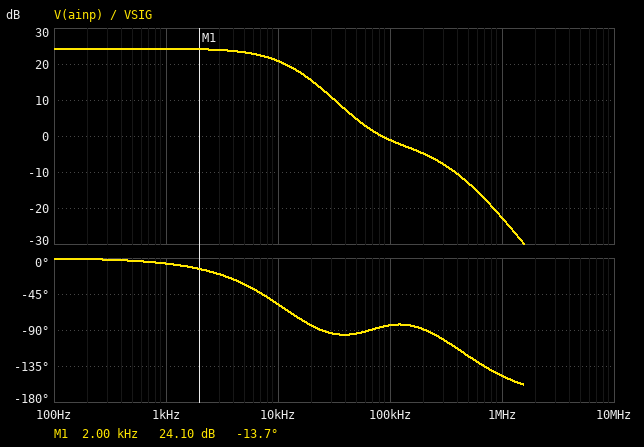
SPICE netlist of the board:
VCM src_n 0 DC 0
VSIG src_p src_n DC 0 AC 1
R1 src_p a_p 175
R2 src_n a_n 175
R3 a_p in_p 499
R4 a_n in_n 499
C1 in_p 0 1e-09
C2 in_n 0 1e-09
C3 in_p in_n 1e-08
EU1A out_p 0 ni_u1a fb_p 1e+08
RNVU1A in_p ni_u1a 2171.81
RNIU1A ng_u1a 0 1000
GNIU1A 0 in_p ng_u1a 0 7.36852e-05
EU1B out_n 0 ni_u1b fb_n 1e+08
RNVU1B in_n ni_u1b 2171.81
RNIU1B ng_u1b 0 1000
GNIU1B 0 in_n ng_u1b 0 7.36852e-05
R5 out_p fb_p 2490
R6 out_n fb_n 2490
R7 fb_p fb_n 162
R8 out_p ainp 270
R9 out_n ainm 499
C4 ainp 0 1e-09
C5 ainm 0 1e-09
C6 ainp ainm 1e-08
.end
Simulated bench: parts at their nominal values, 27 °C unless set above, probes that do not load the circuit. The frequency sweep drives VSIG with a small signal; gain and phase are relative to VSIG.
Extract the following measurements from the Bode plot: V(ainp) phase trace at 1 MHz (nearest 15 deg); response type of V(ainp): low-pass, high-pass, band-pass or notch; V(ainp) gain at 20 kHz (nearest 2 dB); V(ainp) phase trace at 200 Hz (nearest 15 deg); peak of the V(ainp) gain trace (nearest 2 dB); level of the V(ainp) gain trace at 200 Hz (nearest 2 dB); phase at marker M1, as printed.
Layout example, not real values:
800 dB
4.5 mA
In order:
-150 deg
low-pass
16 dB
0 deg
24 dB
24 dB
-13.7 deg
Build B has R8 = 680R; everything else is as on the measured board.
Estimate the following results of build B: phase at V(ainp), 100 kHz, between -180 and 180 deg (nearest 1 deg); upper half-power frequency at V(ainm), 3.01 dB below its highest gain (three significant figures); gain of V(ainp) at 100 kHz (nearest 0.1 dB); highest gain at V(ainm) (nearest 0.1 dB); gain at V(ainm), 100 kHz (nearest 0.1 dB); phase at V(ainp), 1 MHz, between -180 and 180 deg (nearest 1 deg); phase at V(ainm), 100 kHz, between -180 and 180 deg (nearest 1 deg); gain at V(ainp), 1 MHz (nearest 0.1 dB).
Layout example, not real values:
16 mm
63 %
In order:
-38 deg
7.92 kHz
-16.2 dB
23.7 dB
-4.9 dB
-150 deg
1 deg
-31.9 dB
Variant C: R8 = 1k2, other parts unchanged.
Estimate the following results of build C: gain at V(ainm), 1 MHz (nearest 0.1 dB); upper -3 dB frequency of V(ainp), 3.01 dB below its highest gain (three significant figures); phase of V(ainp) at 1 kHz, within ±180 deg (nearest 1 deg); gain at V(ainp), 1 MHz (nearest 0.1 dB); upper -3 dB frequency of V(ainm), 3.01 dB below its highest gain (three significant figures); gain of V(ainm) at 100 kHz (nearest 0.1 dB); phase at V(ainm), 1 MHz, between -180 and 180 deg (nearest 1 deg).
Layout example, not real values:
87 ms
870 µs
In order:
-40.7 dB
6.48 kHz
-14 deg
-39.1 dB
7.04 kHz
-3.1 dB
-127 deg
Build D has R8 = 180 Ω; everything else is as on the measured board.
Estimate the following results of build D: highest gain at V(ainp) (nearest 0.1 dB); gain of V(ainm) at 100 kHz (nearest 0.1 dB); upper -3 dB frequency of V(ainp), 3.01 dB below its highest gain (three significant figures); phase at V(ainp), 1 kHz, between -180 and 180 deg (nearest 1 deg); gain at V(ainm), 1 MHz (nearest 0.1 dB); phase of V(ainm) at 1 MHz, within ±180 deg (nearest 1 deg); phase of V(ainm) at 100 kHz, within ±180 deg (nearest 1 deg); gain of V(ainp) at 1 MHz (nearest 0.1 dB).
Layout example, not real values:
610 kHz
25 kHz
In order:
24.3 dB
1.8 dB
9.75 kHz
-6 deg
-20.3 dB
-139 deg
-46 deg
-19.4 dB
